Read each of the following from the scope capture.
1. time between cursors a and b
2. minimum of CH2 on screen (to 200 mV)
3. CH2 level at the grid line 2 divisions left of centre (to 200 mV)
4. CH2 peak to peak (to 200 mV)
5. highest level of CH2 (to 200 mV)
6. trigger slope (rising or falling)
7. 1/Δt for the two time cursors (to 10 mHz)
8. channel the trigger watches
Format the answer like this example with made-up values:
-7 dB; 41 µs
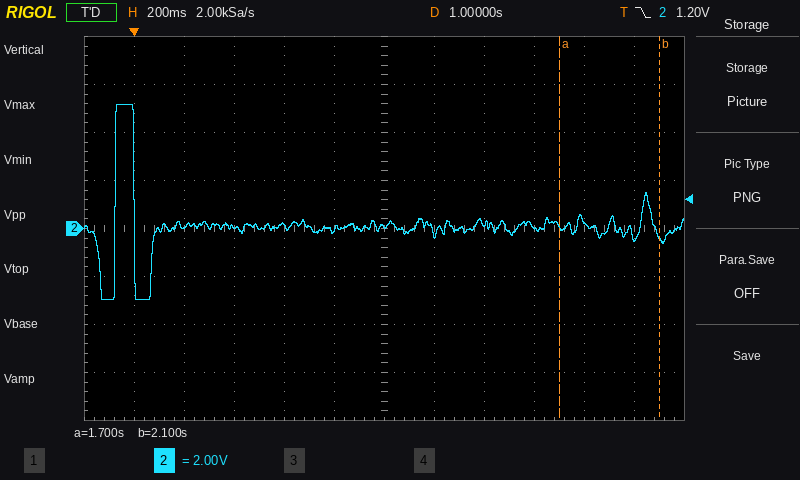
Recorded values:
400 ms; -3.0 V; 0.0 V; 8.2 V; 5.2 V; falling; 2.50 Hz; CH2
